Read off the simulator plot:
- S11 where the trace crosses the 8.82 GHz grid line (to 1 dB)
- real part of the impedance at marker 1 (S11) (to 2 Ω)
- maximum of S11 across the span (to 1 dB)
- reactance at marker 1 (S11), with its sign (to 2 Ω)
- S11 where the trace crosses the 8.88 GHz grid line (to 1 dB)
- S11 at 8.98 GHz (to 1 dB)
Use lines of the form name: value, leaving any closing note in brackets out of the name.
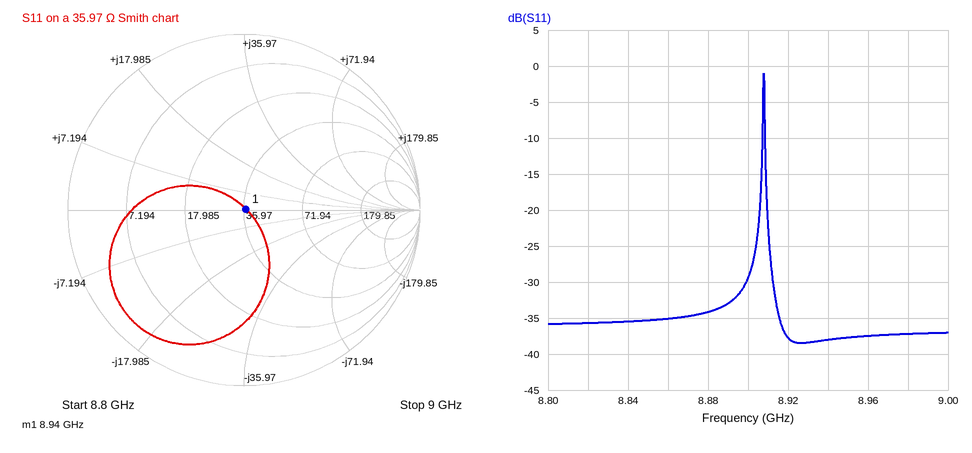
S11 where the trace crosses the 8.82 GHz grid line: -36 dB
real part of the impedance at marker 1 (S11): 36 Ω
maximum of S11 across the span: -1 dB
reactance at marker 1 (S11), with its sign: 0 Ω
S11 where the trace crosses the 8.88 GHz grid line: -34 dB
S11 at 8.98 GHz: -37 dB
